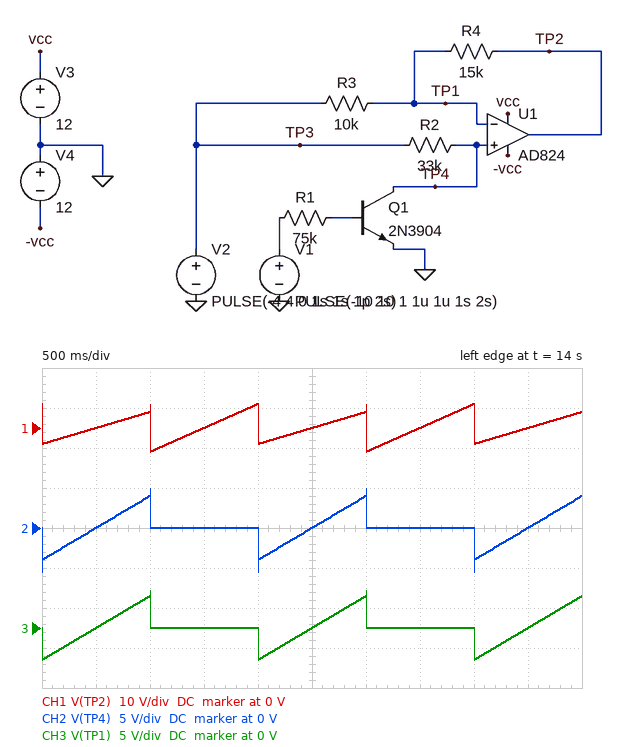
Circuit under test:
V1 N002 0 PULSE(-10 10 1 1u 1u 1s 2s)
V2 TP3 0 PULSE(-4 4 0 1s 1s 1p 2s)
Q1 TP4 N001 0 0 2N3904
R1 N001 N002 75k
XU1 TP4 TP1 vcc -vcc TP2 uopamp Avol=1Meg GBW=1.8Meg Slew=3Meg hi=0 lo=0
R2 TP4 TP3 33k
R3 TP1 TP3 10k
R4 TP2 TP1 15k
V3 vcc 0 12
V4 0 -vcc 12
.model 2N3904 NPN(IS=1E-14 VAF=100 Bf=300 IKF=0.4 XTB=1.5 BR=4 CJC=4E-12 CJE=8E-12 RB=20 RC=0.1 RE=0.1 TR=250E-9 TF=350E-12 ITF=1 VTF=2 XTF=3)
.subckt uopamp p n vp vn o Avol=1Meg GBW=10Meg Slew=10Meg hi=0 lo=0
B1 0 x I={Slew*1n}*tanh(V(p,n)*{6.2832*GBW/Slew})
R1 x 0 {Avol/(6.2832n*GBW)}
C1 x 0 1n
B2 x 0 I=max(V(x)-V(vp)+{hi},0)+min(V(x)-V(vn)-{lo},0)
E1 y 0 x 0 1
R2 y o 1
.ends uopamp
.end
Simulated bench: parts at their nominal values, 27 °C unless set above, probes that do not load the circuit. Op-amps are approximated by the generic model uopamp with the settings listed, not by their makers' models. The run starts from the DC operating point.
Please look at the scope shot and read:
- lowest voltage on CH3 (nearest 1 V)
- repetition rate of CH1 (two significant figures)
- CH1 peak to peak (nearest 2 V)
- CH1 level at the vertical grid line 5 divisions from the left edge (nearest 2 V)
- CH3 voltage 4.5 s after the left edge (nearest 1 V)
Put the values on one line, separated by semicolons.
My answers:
-4 V; 1.0 Hz; 12 V; 0 V; 0 V
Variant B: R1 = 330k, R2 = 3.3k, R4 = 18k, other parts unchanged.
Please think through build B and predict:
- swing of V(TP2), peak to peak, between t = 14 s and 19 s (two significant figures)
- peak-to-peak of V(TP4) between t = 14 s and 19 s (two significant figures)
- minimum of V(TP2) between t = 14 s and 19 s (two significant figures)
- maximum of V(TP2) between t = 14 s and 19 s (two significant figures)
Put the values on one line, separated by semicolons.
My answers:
11 V; 8.1 V; -7.0 V; 4.1 V
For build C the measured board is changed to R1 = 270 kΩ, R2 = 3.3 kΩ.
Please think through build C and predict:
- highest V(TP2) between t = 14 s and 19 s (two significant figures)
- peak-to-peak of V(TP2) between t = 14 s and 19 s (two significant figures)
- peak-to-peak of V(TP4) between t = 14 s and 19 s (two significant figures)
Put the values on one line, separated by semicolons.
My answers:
4.1 V; 10 V; 8.1 V
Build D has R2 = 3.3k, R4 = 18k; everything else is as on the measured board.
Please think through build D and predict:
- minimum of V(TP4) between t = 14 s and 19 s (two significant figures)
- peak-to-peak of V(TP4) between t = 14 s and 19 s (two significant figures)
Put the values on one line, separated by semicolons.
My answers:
-4.2 V; 8.3 V
